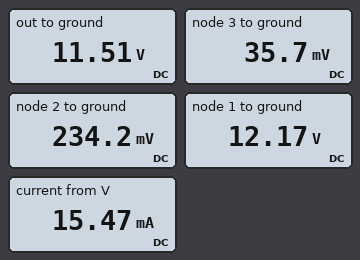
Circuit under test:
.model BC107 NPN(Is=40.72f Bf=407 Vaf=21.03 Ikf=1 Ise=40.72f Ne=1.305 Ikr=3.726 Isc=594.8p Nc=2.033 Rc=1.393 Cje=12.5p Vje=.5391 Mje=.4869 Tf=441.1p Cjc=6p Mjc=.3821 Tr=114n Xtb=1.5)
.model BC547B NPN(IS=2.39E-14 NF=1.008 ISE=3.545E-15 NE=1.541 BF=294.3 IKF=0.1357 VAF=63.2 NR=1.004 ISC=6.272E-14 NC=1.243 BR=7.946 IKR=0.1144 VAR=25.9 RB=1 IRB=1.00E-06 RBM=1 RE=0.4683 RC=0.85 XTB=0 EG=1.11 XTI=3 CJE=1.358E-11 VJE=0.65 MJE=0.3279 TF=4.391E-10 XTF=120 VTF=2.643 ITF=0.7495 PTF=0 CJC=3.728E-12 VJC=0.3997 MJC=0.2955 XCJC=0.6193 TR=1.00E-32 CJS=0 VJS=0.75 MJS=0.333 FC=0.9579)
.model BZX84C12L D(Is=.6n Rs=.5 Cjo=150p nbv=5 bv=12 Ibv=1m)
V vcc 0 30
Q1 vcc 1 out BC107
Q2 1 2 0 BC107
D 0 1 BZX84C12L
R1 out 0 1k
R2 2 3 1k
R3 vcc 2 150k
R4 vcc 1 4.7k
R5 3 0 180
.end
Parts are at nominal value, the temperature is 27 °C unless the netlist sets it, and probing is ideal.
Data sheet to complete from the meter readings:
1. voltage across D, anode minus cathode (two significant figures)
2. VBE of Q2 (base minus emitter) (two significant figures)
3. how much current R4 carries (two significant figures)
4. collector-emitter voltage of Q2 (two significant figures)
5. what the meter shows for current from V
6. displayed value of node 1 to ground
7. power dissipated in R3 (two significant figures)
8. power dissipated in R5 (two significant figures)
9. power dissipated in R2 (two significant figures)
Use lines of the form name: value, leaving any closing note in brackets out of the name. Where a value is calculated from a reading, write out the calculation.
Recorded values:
voltage across D, anode minus cathode: 0 V - 12.17 V = -12 V
VBE of Q2 (base minus emitter): 234.2 mV = 230 mV
how much current R4 carries: (30 V - 12.17 V) / 4.7 kΩ = 3.8 mA
collector-emitter voltage of Q2: 12.17 V = 12 V
what the meter shows for current from V: 15.47 mA
displayed value of node 1 to ground: 12.17 V
power dissipated in R3: (30 V - 234.2 mV)^2 / 150 kΩ = 5.9 mW
power dissipated in R5: (35.7 mV)^2 / 180 Ω = 7.1 µW
power dissipated in R2: (234.2 mV - 35.7 mV)^2 / 1 kΩ = 39 µW
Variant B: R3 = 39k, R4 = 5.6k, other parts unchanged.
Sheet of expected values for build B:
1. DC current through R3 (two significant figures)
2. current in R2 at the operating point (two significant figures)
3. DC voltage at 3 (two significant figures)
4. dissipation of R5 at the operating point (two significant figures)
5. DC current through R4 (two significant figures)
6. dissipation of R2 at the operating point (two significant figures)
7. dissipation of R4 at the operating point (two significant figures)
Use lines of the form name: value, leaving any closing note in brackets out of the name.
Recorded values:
DC current through R3: 750 µA
current in R2 at the operating point: 560 µA
DC voltage at 3: 100 mV
dissipation of R5 at the operating point: 57 µW
DC current through R4: 5.3 mA
dissipation of R2 at the operating point: 320 µW
dissipation of R4 at the operating point: 160 mW
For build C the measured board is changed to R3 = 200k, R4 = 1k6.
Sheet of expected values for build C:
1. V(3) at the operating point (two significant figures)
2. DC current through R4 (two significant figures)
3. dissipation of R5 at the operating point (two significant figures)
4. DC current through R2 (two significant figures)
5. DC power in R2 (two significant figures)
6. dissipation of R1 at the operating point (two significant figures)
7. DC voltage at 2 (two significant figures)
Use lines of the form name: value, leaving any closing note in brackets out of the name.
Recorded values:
V(3) at the operating point: 27 mV
DC current through R4: 11 mA
dissipation of R5 at the operating point: 4.0 µW
DC current through R2: 150 µA
DC power in R2: 22 µW
dissipation of R1 at the operating point: 140 mW
DC voltage at 2: 180 mV
